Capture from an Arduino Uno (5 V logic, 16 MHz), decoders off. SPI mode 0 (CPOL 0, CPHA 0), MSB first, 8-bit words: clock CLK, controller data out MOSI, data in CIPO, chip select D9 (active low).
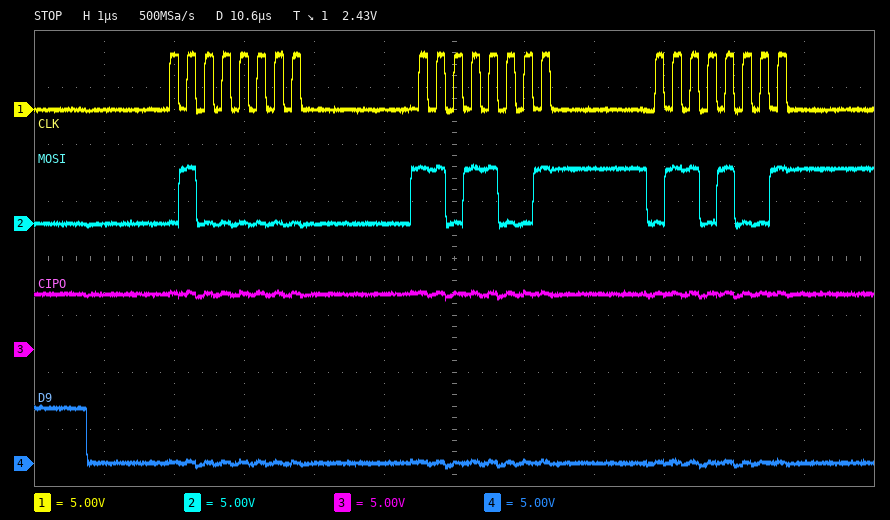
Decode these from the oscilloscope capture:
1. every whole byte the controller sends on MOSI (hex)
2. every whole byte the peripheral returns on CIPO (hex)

40 D9 69
FF FF FF
